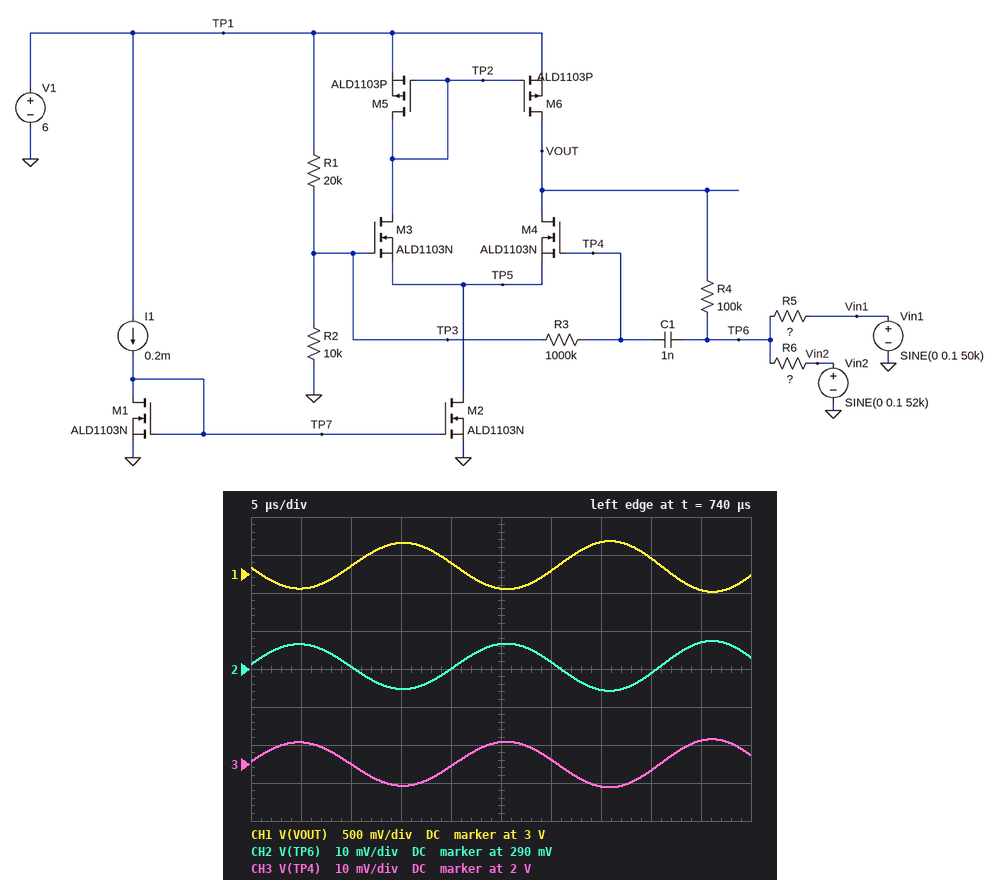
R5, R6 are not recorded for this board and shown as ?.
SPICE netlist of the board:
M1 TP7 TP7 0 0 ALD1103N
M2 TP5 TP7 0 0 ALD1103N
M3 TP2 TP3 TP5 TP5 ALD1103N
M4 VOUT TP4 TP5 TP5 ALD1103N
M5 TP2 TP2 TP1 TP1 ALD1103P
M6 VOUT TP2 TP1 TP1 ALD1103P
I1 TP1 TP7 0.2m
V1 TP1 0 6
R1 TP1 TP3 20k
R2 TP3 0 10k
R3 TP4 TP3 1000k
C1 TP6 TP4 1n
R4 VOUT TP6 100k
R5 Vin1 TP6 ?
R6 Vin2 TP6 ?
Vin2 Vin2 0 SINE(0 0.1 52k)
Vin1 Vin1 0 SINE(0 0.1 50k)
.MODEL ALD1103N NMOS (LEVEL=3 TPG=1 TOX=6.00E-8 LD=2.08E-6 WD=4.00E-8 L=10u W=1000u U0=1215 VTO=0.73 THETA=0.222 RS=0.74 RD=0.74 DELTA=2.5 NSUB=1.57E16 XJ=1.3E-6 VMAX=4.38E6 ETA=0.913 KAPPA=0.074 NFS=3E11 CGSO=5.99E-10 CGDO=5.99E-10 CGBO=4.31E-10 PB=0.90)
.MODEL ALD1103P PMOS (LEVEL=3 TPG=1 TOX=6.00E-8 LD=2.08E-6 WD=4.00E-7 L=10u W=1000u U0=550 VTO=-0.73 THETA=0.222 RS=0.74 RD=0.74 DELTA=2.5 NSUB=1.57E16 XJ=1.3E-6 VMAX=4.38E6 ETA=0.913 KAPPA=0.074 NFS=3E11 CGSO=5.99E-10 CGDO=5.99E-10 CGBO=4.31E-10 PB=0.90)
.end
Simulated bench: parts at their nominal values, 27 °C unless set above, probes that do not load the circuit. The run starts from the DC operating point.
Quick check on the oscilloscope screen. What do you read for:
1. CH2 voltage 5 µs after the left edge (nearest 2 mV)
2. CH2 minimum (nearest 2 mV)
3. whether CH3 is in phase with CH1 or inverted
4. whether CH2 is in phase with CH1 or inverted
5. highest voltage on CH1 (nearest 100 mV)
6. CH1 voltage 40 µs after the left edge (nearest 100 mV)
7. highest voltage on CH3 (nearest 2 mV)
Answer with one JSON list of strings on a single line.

["296 mV", "284 mV", "inverted", "inverted", "3.4 V", "3.2 V", "2.006 V"]
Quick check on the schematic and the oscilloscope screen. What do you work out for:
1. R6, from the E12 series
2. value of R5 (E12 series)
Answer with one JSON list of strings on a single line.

["33 kΩ", "15 kΩ"]
